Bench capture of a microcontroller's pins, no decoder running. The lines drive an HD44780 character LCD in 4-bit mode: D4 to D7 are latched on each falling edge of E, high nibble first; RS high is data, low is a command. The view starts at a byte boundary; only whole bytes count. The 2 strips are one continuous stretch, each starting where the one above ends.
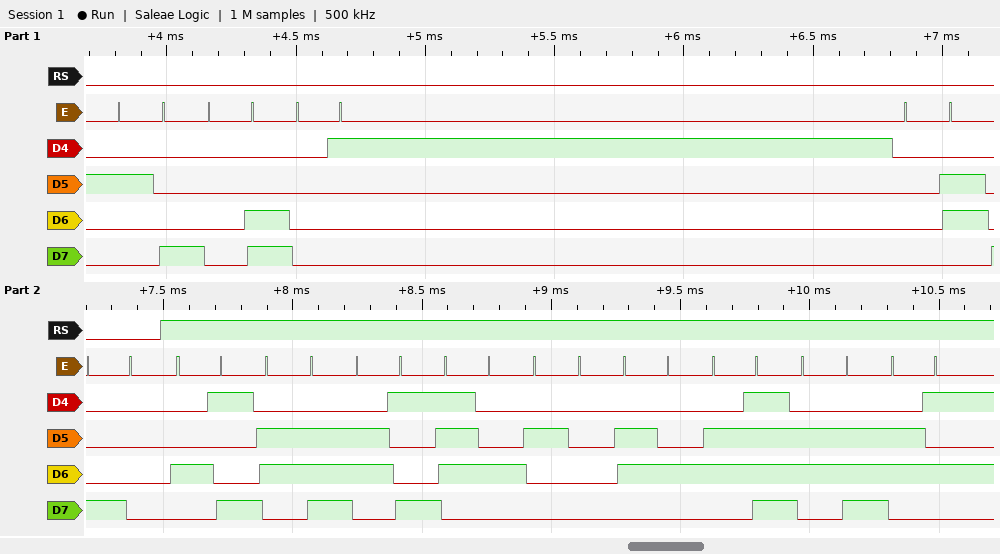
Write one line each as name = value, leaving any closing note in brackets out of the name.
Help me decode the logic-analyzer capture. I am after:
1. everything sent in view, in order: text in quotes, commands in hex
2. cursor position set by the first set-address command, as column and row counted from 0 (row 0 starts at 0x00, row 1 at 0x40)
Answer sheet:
everything sent in view, in order: text in quotes, commands in hex = 0x28 0x0C 0x01 0x06 0x80 "Init done"
cursor position set by the first set-address command, as column and row counted from 0 = column 0, row 0
